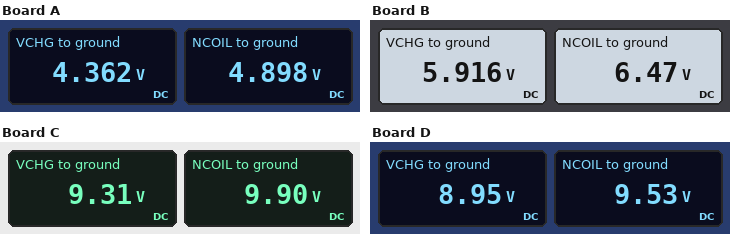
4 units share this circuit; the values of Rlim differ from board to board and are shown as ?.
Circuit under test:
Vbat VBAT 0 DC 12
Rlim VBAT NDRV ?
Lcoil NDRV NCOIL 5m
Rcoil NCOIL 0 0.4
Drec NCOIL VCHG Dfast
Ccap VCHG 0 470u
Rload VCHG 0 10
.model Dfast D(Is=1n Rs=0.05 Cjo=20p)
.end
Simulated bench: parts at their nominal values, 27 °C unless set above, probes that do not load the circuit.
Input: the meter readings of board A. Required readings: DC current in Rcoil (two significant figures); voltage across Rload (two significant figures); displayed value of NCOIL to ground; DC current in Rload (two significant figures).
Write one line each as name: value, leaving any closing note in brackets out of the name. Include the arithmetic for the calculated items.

DC current in Rcoil: (4.898 V) / 400 mΩ = 12 A
voltage across Rload: 4.362 V = 4.4 V
displayed value of NCOIL to ground: 4.898 V
DC current in Rload: (4.362 V) / 10 Ω = 440 mA
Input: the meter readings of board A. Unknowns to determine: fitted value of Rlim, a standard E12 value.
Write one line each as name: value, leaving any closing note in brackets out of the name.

fitted value of Rlim, a standard E12 value: 0.56 Ω
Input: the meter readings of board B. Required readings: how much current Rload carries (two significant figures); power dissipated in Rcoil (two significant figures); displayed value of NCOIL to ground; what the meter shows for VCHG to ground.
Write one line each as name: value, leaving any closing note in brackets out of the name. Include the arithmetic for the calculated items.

how much current Rload carries: (5.916 V) / 10 Ω = 590 mA
power dissipated in Rcoil: (6.47 V)^2 / 400 mΩ = 100 W
displayed value of NCOIL to ground: 6.47 V
what the meter shows for VCHG to ground: 5.916 V
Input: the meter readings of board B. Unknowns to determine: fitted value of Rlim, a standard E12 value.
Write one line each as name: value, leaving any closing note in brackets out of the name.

fitted value of Rlim, a standard E12 value: 0.33 Ω
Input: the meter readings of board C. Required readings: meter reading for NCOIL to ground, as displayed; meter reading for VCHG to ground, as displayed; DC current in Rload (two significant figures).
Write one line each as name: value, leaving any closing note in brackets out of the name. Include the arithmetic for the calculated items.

meter reading for NCOIL to ground, as displayed: 9.90 V
meter reading for VCHG to ground, as displayed: 9.31 V
DC current in Rload: (9.31 V) / 10 Ω = 930 mA
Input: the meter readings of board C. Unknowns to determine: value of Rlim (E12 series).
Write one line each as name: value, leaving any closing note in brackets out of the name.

value of Rlim: 0.082 Ω
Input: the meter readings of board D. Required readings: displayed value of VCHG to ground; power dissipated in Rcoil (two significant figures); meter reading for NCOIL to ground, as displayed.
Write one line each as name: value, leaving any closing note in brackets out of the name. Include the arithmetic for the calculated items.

displayed value of VCHG to ground: 8.95 V
power dissipated in Rcoil: (9.53 V)^2 / 400 mΩ = 230 W
meter reading for NCOIL to ground, as displayed: 9.53 V
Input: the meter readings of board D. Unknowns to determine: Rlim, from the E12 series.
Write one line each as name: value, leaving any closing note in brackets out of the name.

Rlim, from the E12 series: 0.1 Ω
